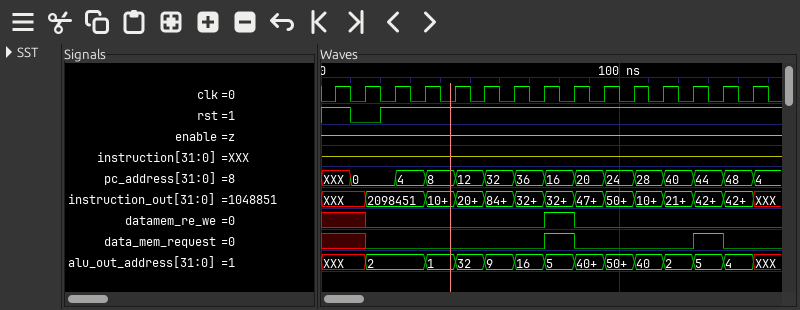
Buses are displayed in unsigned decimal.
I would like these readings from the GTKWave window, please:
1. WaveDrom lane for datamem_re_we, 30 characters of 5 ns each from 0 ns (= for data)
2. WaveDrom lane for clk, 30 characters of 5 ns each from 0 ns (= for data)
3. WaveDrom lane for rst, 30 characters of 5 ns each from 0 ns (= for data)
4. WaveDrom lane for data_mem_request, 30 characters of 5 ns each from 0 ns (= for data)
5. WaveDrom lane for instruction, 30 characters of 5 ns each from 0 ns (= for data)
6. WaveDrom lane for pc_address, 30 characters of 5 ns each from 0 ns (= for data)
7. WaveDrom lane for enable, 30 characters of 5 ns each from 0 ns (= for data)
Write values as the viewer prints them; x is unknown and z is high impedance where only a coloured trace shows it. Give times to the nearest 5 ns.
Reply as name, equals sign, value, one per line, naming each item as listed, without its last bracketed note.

WaveDrom lane for datamem_re_we, 30 characters of 5 ns each from 0 ns = {name: 'datamem_re_we', wave: 'x..0...........1.0............'}
WaveDrom lane for clk, 30 characters of 5 ns each from 0 ns = {name: 'clk', wave: '010101010101010101010101010101'}
WaveDrom lane for rst, 30 characters of 5 ns each from 0 ns = {name: 'rst', wave: '1.0.1.........................'}
WaveDrom lane for data_mem_request, 30 characters of 5 ns each from 0 ns = {name: 'data_mem_request', wave: 'x..0...........1.0.......1.0..'}
WaveDrom lane for instruction, 30 characters of 5 ns each from 0 ns = {name: 'instruction', wave: 'z.............................'}
WaveDrom lane for pc_address, 30 characters of 5 ns each from 0 ns = {name: 'pc_address', wave: 'x.=..=.=.=.=.=.=.=.=.=.=.=.=.=', data: '0 4 8 12 32 36 16 20 24 28 40 44 48 4'}
WaveDrom lane for enable, 30 characters of 5 ns each from 0 ns = {name: 'enable', wave: 'z.............................'}
